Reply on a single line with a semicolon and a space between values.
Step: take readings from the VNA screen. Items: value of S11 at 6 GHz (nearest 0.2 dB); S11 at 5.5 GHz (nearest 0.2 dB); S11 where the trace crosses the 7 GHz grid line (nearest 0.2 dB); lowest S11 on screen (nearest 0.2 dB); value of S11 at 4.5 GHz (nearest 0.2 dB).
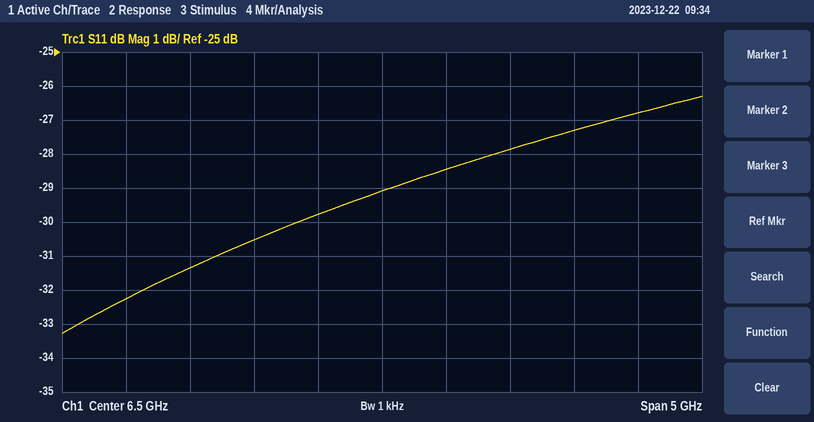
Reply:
-29.8 dB; -30.6 dB; -28.4 dB; -33.2 dB; -32.2 dB
